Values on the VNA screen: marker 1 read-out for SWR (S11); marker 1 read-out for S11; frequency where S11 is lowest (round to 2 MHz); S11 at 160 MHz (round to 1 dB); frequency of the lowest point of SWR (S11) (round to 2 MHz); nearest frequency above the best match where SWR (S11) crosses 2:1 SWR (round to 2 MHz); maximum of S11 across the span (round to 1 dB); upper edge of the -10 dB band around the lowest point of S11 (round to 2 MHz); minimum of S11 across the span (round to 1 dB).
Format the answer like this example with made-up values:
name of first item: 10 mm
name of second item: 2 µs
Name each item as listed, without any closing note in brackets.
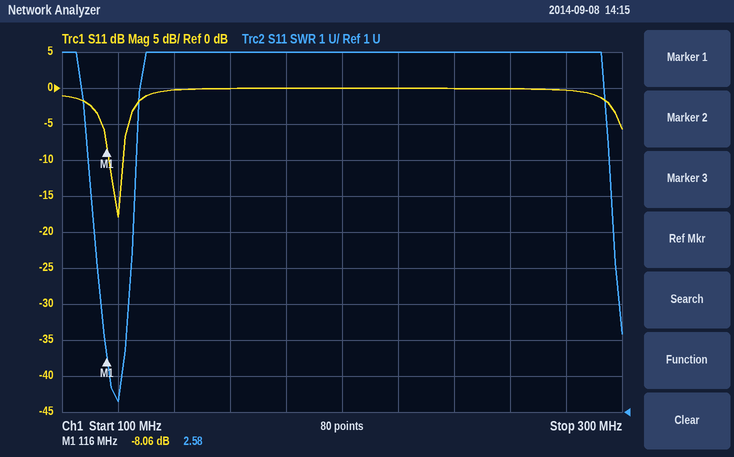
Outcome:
marker 1 read-out for SWR: 2.58
marker 1 read-out for S11: -8.06 dB
frequency where S11 is lowest: 120 MHz
S11 at 160 MHz: 0 dB
frequency of the lowest point of SWR (S11): 120 MHz
nearest frequency above the best match where SWR (S11) crosses 2:1 SWR: 122 MHz
maximum of S11 across the span: 0 dB
upper edge of the -10 dB band around the lowest point of S11: 122 MHz
minimum of S11 across the span: -18 dB
